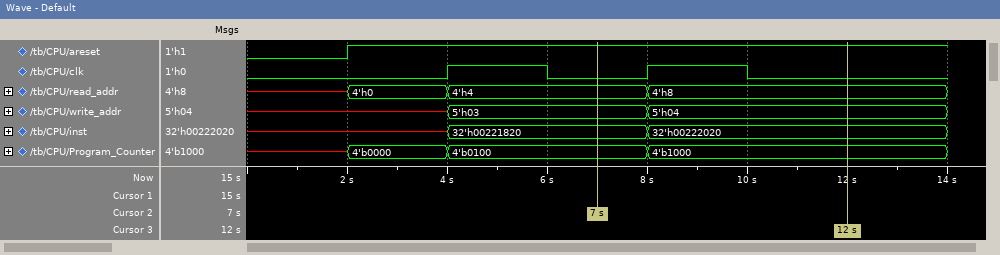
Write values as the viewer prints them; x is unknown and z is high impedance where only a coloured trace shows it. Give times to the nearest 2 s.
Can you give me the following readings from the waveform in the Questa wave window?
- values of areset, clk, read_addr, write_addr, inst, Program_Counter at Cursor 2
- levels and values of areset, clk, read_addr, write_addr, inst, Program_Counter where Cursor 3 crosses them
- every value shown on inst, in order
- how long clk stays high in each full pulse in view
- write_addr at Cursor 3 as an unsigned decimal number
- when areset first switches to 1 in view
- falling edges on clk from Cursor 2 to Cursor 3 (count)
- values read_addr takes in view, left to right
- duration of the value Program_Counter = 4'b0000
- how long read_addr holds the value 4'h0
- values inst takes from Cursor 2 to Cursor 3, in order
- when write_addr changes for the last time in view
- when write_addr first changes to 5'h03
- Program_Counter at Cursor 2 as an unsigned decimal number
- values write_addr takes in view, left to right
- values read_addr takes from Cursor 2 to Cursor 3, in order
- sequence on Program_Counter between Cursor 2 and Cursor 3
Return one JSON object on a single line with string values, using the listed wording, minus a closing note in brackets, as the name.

{"values of areset, clk, read_addr, write_addr, inst, Program_Counter at Cursor 2": "areset=1, clk=0, read_addr=4'h4, write_addr=5'h03, inst=32'h00221820, Program_Counter=4'b0100", "levels and values of areset, clk, read_addr, write_addr, inst, Program_Counter where Cursor 3 crosses them": "areset=1, clk=0, read_addr=4'h8, write_addr=5'h04, inst=32'h00222020, Program_Counter=4'b1000", "every value shown on inst, in order": "x, 32'h00221820, 32'h00222020", "how long clk stays high in each full pulse in view": "2 s, 2 s", "write_addr at Cursor 3 as an unsigned decimal number": "4", "when areset first switches to 1 in view": "2 s", "falling edges on clk from Cursor 2 to Cursor 3": "1", "values read_addr takes in view, left to right": "x, 4'h0, 4'h4, 4'h8", "duration of the value Program_Counter = 4'b0000": "2 s", "how long read_addr holds the value 4'h0": "2 s", "values inst takes from Cursor 2 to Cursor 3, in order": "32'h00221820, 32'h00222020", "when write_addr changes for the last time in view": "8 s", "when write_addr first changes to 5'h03": "4 s", "Program_Counter at Cursor 2 as an unsigned decimal number": "4", "values write_addr takes in view, left to right": "x, 5'h03, 5'h04", "values read_addr takes from Cursor 2 to Cursor 3, in order": "4'h4, 4'h8", "sequence on Program_Counter between Cursor 2 and Cursor 3": "4'b0100, 4'b1000"}
